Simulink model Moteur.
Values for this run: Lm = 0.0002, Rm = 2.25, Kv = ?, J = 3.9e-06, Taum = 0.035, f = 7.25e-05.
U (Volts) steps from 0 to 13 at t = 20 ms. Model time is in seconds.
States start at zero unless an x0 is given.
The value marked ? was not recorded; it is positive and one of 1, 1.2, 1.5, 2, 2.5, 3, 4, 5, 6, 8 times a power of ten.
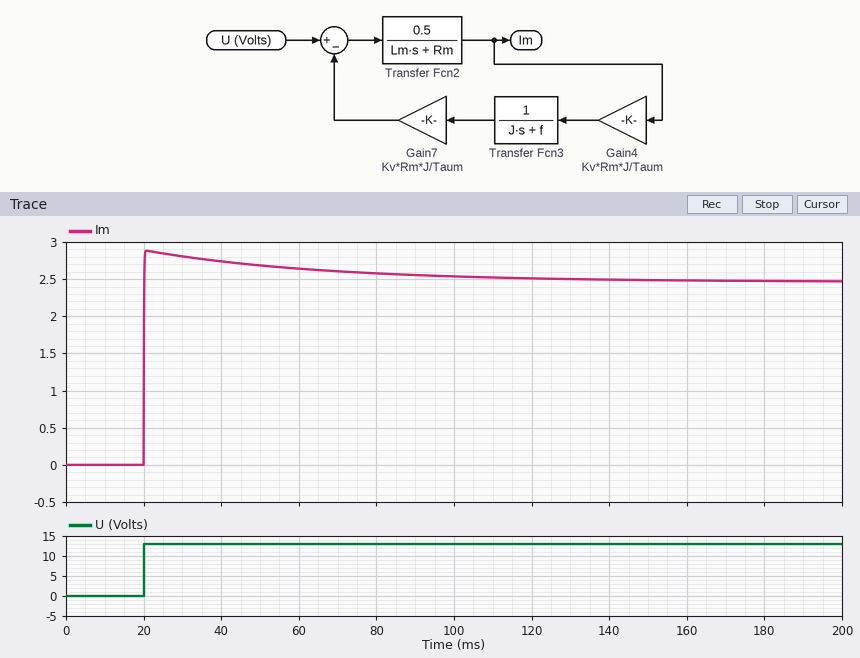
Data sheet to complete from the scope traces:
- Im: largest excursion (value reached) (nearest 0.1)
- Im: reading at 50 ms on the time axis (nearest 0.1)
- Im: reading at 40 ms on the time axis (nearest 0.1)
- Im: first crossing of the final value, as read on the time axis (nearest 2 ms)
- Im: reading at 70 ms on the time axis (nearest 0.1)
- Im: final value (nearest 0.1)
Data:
2.9
2.7
2.7
20 ms
2.6
2.5
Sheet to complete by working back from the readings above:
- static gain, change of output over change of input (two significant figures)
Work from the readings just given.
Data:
0.19
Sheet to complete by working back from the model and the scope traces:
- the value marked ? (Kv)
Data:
30
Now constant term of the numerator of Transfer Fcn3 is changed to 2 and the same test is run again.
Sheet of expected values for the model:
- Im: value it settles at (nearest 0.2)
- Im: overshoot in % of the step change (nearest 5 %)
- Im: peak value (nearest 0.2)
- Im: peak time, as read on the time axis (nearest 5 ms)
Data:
2.2
35 %
2.8
20 ms
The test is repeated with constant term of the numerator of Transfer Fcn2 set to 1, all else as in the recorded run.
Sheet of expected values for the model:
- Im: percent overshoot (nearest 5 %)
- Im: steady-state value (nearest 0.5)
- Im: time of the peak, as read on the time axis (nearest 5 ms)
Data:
35 %
4.5
20 ms
